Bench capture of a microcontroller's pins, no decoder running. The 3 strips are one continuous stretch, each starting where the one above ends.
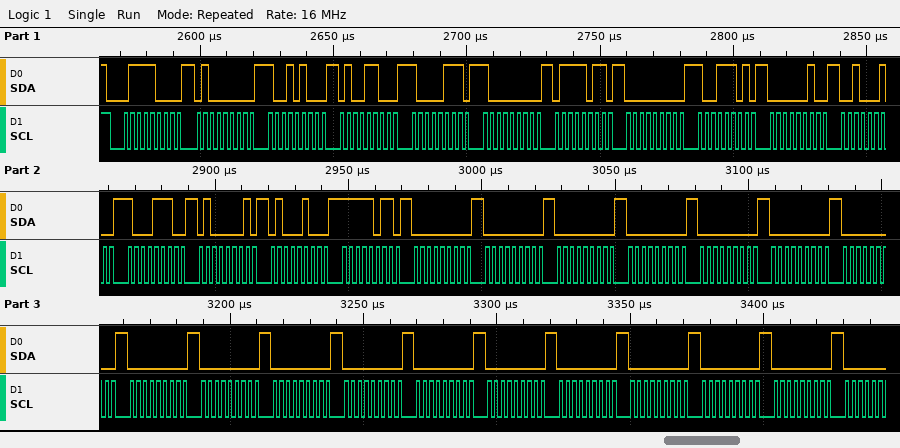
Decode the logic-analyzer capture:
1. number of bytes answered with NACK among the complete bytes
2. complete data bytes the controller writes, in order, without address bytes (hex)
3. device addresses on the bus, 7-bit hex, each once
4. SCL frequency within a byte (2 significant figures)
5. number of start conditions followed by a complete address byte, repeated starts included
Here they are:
0
40 94 4C 87 80 7B 00 9D 02 22 8E 41 44 FB 00 00 00 00 00 00 00 00 00 00 00 00 00 00 00 00 00
0x3C
400 kHz
1
